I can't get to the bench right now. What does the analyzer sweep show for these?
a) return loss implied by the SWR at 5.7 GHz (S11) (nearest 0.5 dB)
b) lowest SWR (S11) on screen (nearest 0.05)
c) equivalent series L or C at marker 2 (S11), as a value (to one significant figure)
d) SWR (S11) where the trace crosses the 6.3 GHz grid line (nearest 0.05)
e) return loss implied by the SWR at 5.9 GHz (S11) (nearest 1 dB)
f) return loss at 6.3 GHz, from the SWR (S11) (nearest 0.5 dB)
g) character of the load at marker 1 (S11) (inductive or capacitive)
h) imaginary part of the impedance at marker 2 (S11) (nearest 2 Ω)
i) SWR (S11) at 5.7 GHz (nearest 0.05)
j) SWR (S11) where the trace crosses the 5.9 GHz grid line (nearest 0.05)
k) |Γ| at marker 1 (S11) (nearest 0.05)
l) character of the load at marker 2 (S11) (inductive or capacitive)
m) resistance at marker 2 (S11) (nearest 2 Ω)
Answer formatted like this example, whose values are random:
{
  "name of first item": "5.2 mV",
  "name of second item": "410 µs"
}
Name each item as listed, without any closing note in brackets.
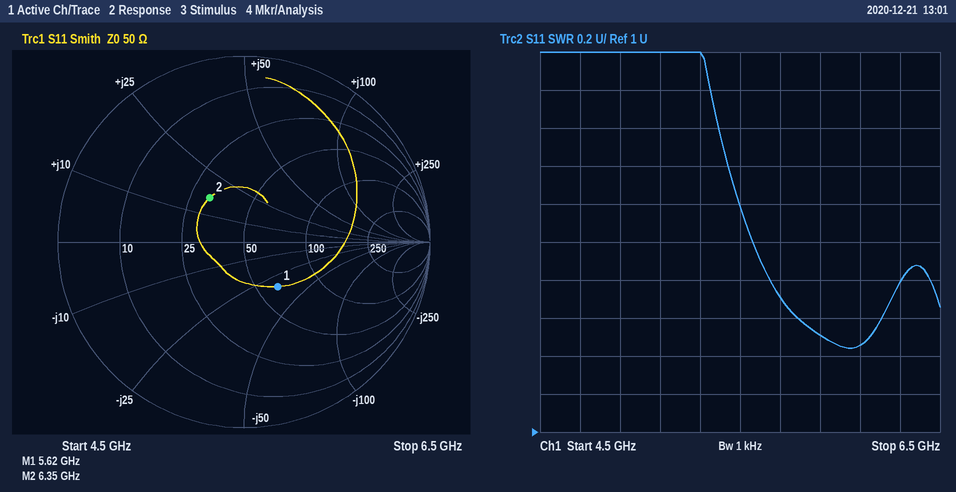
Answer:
{
  "return loss implied by the SWR at 5.7 GHz (S11)": "11.5 dB",
  "lowest SWR (S11) on screen": "1.45",
  "equivalent series L or C at marker 2 (S11), as a value": "400 pH",
  "SWR (S11) where the trace crosses the 6.3 GHz grid line": "1.80",
  "return loss implied by the SWR at 5.9 GHz (S11)": "14 dB",
  "return loss at 6.3 GHz, from the SWR (S11)": "11.0 dB",
  "character of the load at marker 1 (S11)": "capacitive",
  "imaginary part of the impedance at marker 2 (S11)": "+16 Ω",
  "SWR (S11) at 5.7 GHz": "1.70",
  "SWR (S11) where the trace crosses the 5.9 GHz grid line": "1.50",
  "|Γ| at marker 1 (S11)": "0.30",
  "character of the load at marker 2 (S11)": "inductive",
  "resistance at marker 2 (S11)": "32 Ω"
}
